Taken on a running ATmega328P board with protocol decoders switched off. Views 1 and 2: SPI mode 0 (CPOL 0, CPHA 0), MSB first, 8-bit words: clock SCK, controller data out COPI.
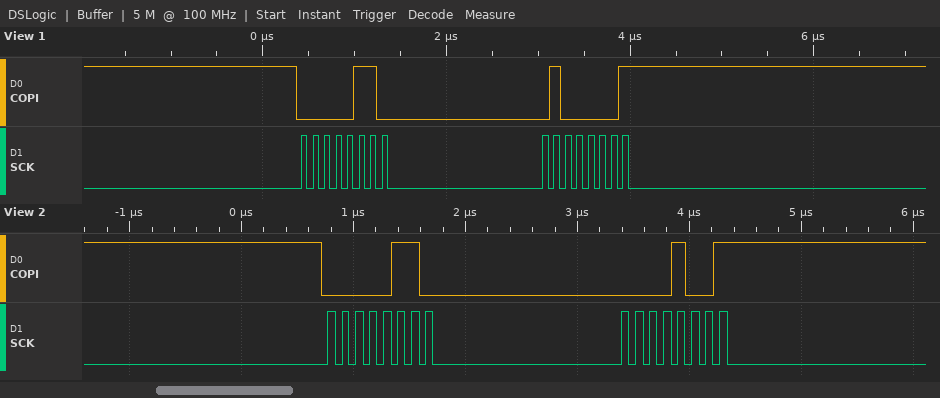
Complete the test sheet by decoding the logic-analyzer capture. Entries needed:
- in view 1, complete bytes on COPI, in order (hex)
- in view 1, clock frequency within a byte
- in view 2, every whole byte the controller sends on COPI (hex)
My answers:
06 41
8 MHz
0x06 0x09
